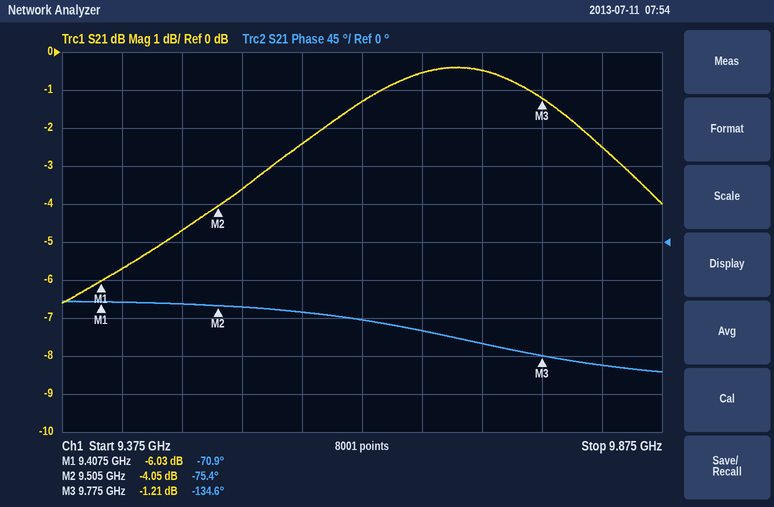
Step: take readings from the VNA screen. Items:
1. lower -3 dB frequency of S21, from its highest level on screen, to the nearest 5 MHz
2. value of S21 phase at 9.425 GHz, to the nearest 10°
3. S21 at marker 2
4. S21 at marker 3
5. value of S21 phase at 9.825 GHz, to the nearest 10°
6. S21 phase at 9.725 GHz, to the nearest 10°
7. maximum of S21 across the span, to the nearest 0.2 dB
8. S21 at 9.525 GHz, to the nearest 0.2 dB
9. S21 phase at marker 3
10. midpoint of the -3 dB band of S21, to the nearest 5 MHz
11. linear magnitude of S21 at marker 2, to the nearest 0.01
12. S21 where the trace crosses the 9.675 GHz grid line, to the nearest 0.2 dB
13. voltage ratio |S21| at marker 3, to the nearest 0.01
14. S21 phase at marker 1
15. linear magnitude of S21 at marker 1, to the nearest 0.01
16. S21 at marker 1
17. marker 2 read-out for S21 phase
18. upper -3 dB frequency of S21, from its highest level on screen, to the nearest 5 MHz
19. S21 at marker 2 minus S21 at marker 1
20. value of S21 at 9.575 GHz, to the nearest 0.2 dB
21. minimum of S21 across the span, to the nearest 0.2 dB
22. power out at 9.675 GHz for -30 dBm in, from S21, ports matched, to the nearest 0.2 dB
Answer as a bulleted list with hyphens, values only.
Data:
- 9.535 GHz
- -70°
- -4.05 dB
- -1.21 dB
- -150°
- -120°
- -0.4 dB
- -3.6 dB
- -134.6°
- 9.695 GHz
- 0.63
- -0.6 dB
- 0.87
- -70.9°
- 0.50
- -6.03 dB
- -75.4°
- 9.855 GHz
- 1.98 dB
- -2.4 dB
- -6.6 dB
- -30.6 dBm
